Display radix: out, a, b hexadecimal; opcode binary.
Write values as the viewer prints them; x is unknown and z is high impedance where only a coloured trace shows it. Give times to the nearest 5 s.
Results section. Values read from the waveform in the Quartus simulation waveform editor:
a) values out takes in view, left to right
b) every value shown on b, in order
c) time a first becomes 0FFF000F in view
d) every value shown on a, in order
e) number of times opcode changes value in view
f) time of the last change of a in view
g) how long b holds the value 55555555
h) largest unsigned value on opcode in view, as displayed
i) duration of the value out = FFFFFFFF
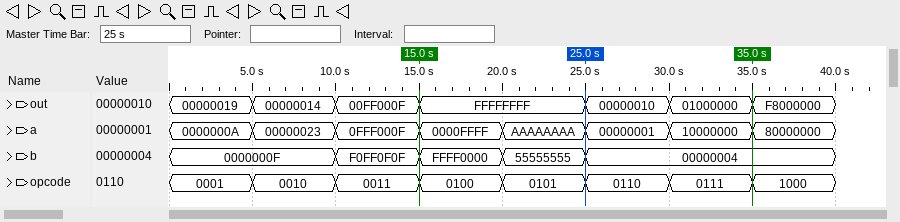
00000019, 00000014, 00FF000F, FFFFFFFF, 00000010, 01000000, F8000000
0000000F, F0FF0F0F, FFFF0000, 55555555, 00000004
10 s
0000000A, 00000023, 0FFF000F, 0000FFFF, AAAAAAAA, 00000001, 10000000, 80000000
7
35 s
5 s
1000
10 s
